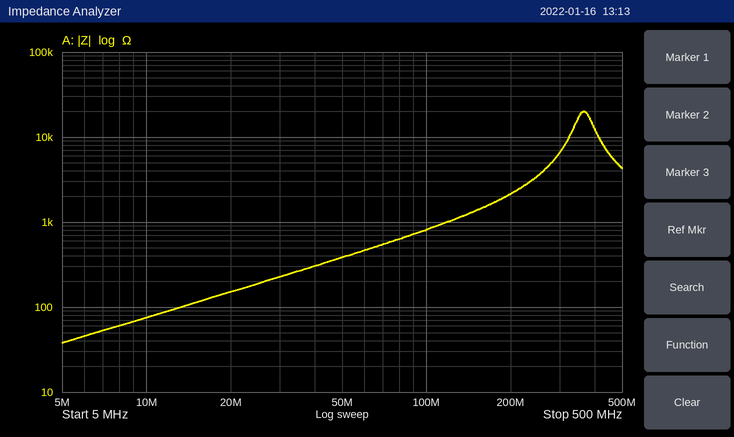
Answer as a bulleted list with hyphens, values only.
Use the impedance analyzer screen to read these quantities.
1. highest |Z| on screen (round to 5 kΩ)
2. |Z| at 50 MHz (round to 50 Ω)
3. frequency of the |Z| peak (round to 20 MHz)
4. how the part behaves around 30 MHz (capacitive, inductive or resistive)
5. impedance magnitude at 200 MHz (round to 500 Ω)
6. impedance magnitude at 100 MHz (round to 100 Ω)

- 20 kΩ
- 400 Ω
- 360 MHz
- inductive
- 2.0 kΩ
- 800 Ω
